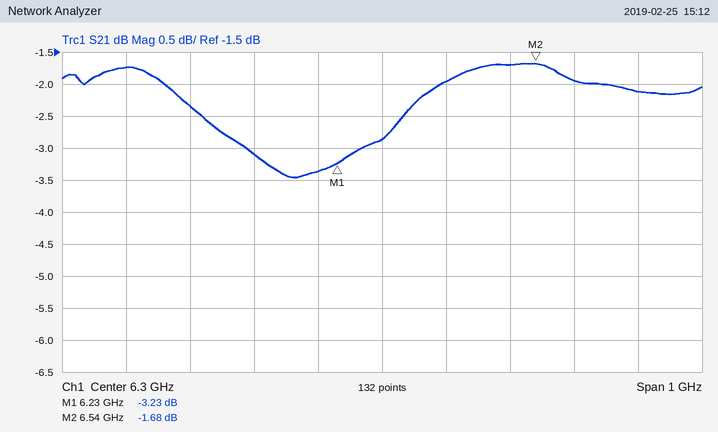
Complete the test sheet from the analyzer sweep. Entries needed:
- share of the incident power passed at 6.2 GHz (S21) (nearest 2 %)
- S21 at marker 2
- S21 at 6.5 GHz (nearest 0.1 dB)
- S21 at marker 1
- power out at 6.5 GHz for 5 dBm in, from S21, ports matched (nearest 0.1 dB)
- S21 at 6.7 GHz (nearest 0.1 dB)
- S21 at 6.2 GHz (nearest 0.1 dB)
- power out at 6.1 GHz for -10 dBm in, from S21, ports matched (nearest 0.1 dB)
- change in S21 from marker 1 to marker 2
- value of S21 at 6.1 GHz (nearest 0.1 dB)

46 %
-1.68 dB
-1.7 dB
-3.23 dB
3.3 dBm
-2.1 dB
-3.4 dB
-13.1 dBm
1.55 dB
-3.1 dB
